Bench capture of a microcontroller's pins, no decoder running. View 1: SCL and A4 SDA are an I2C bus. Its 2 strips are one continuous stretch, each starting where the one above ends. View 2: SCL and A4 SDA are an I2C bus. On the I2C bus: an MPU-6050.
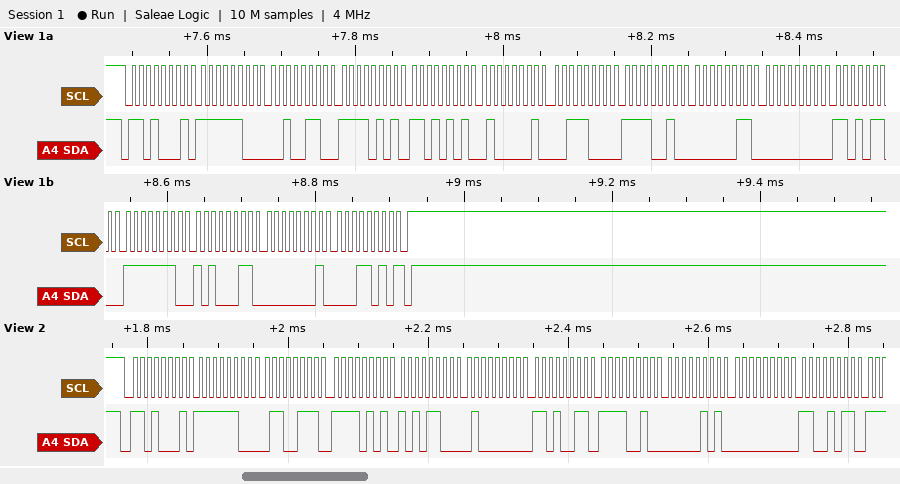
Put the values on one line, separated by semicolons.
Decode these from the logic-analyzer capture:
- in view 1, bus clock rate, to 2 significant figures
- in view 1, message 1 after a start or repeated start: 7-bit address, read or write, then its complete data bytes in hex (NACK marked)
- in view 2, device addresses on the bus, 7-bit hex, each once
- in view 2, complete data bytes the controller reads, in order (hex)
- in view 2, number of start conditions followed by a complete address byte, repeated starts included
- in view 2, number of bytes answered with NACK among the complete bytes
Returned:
100 kHz; 0x68 read: FC 26 F5 D5 41 38 F2 03 00 D6 FE A3 01 1A NACK; 0x68; FC 67 F5 AC 40 D3 F2 05 00 CB; 1; 0
